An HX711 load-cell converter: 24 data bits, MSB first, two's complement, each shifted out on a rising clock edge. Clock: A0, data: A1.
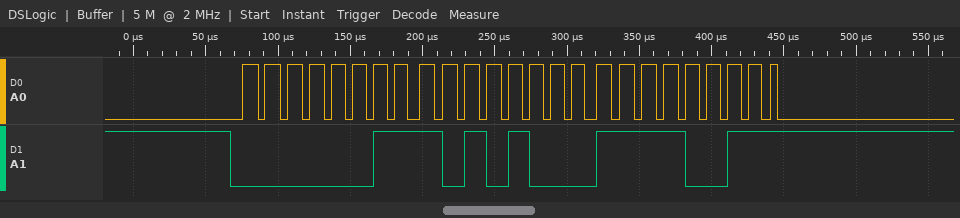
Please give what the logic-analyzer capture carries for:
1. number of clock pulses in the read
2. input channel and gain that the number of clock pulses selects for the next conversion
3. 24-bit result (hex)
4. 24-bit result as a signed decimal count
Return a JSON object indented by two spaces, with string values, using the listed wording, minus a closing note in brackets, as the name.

{
  "number of clock pulses in the read": "25",
  "input channel and gain that the number of clock pulses selects for the next conversion": "channel A, gain 128",
  "24-bit result": "0x03A8F3",
  "24-bit result as a signed decimal count": "239859"
}
